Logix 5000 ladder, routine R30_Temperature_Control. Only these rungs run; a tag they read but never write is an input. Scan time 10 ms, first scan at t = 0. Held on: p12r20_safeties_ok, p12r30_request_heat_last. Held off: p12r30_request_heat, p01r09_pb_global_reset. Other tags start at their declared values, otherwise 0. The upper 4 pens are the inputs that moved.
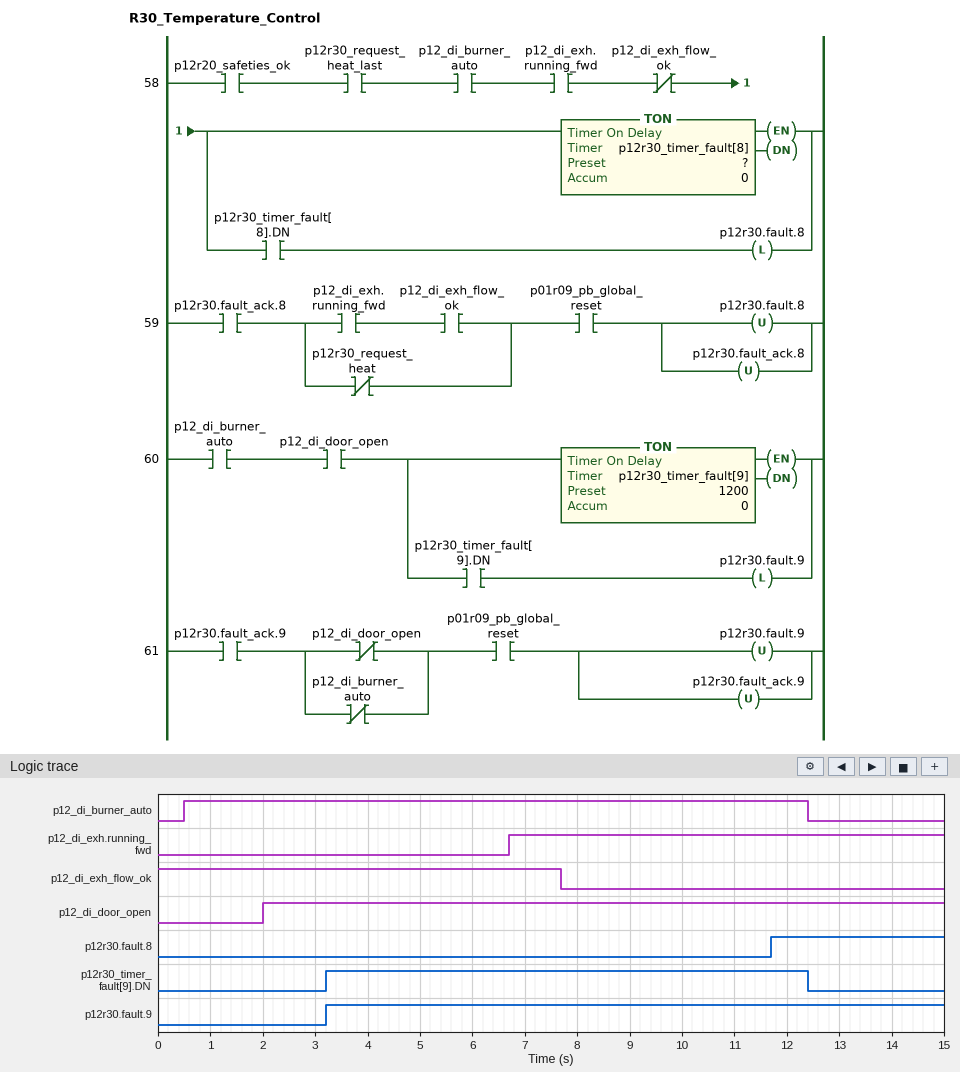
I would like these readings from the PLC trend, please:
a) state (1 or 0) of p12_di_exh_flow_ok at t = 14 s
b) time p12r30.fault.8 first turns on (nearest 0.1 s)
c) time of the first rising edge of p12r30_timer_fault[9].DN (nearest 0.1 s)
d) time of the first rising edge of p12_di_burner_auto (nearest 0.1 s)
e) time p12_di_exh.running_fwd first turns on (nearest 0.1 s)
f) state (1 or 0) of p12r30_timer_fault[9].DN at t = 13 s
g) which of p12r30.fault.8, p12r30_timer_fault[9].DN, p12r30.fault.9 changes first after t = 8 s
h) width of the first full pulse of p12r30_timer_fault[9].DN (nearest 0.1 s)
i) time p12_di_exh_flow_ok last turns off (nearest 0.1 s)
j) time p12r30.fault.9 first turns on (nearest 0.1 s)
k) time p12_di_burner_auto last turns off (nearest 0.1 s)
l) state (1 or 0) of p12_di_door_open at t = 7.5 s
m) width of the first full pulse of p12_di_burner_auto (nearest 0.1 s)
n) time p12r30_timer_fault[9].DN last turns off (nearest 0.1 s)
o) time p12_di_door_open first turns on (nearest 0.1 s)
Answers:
0
11.7 s
3.2 s
0.5 s
6.7 s
0
p12r30.fault.8
9.2 s
7.7 s
3.2 s
12.4 s
1
11.9 s
12.4 s
2.0 s
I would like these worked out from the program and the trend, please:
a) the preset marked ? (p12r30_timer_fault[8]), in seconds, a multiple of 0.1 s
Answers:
4.0 s
